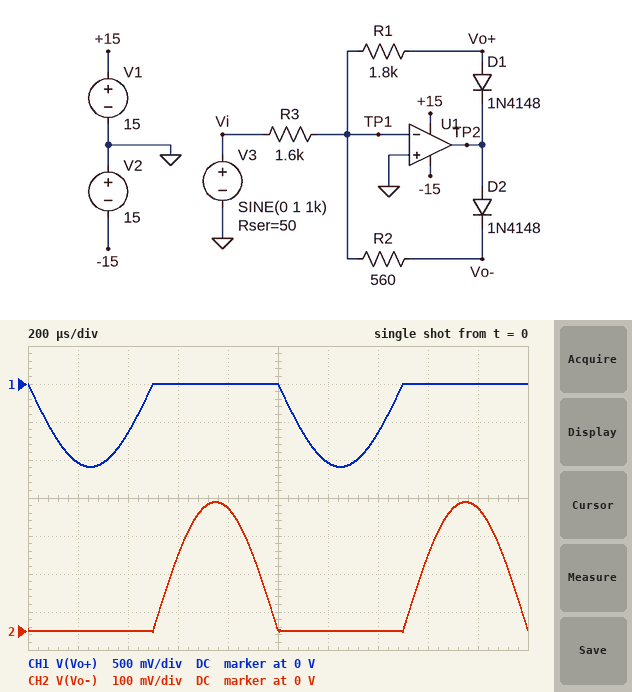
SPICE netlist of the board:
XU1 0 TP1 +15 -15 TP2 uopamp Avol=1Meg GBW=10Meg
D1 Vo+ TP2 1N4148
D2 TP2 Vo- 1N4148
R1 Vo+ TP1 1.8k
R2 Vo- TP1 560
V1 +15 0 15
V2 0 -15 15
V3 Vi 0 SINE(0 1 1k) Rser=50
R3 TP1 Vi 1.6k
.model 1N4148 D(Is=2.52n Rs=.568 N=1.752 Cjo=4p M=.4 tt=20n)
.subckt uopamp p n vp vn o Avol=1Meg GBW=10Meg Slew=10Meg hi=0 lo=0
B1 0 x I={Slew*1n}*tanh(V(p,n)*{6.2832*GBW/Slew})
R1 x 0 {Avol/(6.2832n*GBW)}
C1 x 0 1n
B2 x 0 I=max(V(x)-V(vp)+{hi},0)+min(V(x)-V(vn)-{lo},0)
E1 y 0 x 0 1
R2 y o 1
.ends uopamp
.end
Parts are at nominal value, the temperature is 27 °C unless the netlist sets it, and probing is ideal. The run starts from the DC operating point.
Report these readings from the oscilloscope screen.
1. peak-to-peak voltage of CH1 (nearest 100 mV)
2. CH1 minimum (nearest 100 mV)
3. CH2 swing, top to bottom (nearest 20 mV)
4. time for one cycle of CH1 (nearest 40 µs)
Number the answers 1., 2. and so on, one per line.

1. 1.1 V
2. -1.1 V
3. 340 mV
4. 1.00 ms
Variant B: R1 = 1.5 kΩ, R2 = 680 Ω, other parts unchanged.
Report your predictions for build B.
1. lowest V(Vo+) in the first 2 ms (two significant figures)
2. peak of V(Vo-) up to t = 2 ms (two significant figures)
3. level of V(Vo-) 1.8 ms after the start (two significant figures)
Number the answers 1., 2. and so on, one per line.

1. -910 mV
2. 410 mV
3. 390 mV
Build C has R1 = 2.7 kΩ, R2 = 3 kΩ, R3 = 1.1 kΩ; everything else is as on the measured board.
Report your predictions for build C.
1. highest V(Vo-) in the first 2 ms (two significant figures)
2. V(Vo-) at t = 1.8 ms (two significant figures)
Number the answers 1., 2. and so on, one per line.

1. 2.6 V
2. 2.5 V
